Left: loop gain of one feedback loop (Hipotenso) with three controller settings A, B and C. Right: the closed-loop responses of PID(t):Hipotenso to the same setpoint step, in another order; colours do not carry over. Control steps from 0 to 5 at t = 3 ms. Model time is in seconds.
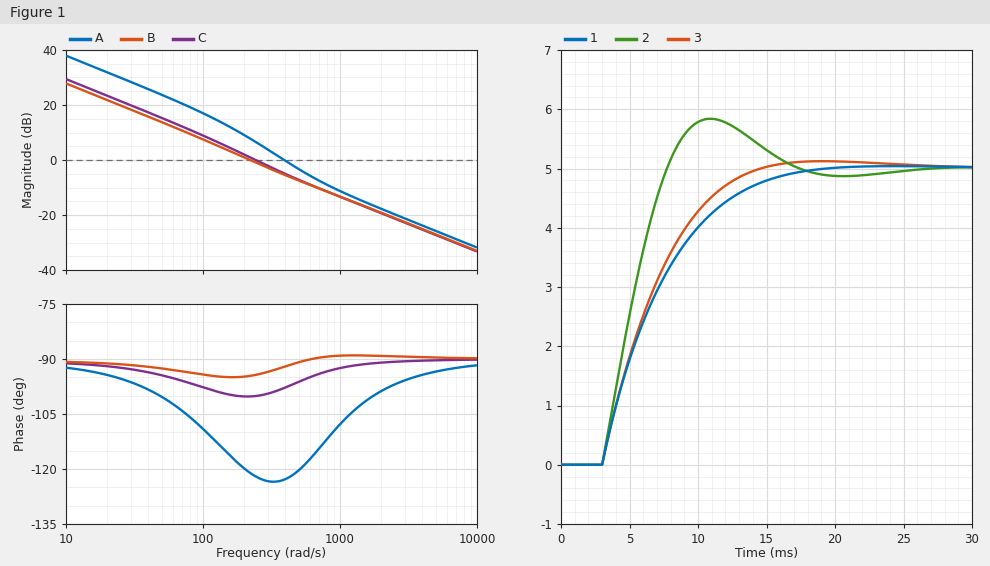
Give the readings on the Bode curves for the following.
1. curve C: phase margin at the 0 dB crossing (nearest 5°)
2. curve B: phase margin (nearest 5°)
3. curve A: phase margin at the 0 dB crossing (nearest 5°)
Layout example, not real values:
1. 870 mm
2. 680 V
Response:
1. 80°
2. 85°
3. 55°
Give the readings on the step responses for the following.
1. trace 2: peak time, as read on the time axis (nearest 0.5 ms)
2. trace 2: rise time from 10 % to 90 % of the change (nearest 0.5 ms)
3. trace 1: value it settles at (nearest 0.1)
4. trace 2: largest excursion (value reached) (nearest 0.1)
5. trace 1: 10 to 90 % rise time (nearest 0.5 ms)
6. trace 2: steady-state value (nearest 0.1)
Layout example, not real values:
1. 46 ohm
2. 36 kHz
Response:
1. 11.0 ms
2. 3.5 ms
3. 5.0
4. 5.8
5. 9.0 ms
6. 5.0
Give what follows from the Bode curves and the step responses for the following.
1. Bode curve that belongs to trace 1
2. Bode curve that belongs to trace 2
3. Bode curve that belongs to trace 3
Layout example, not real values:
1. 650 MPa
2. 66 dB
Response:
1. B
2. A
3. C
